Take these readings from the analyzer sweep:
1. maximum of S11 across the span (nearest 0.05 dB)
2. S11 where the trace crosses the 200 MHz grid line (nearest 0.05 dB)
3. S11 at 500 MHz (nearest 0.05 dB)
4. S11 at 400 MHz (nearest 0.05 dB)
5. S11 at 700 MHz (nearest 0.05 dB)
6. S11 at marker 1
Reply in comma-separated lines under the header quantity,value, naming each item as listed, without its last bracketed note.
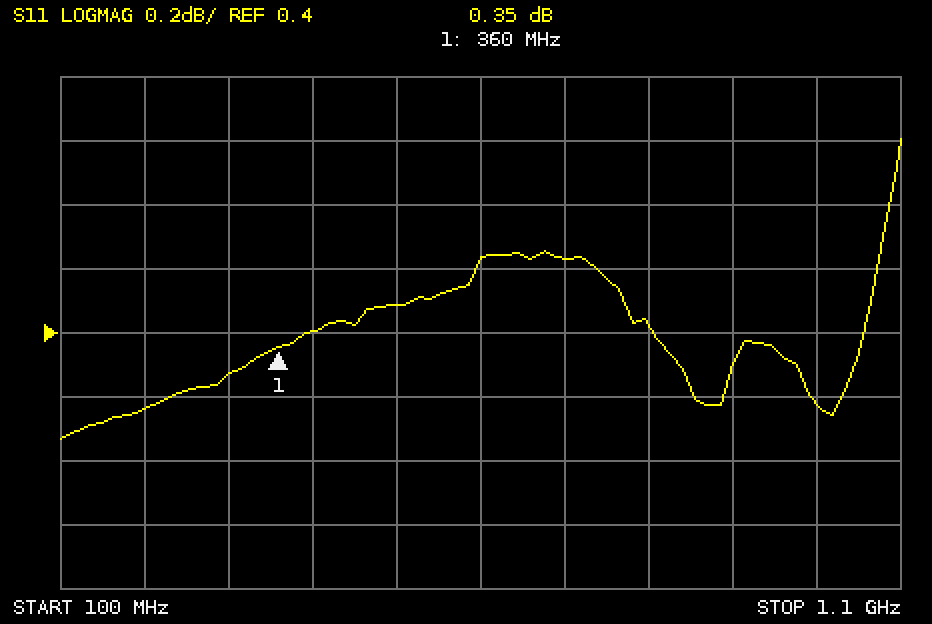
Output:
quantity,value
maximum of S11 across the span,1.00 dB
S11 where the trace crosses the 200 MHz grid line,0.15 dB
S11 at 500 MHz,0.50 dB
S11 at 400 MHz,0.40 dB
S11 at 700 MHz,0.65 dB
S11 at marker 1,0.35 dB
